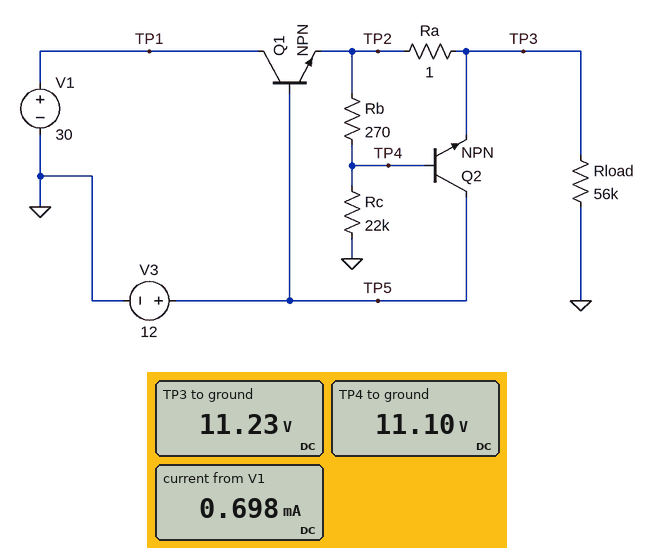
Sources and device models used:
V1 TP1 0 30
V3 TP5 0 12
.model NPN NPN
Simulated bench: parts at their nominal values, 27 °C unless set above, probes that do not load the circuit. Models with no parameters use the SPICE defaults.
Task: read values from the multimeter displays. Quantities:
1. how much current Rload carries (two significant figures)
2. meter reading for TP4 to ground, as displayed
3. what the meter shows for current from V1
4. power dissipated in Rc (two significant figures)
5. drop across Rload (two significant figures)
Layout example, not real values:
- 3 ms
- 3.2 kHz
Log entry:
- 200 µA
- 11.10 V
- 0.698 mA
- 5.6 mW
- 11 V
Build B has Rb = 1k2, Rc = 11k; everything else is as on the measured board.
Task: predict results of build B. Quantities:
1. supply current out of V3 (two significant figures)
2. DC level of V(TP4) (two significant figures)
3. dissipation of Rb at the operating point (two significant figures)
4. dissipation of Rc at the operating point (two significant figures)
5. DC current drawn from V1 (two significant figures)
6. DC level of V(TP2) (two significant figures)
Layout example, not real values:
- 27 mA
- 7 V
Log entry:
- 11 µA
- 10 V
- 1.0 mW
- 9.3 mW
- 1.1 mA
- 11 V
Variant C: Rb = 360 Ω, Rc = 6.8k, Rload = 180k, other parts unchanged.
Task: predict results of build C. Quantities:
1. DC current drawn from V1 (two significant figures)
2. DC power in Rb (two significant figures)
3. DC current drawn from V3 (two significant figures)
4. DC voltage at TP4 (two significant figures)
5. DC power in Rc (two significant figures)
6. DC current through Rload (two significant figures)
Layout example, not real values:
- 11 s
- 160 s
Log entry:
- 1.6 mA
- 880 µW
- 16 µA
- 11 V
- 17 mW
- 62 µA
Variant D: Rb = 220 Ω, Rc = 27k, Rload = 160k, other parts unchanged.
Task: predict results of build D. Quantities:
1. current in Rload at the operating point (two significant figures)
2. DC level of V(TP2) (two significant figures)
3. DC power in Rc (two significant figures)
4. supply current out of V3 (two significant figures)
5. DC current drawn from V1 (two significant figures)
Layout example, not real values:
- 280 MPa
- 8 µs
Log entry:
- 70 µA
- 11 V
- 4.6 mW
- 4.8 µA
- 480 µA
